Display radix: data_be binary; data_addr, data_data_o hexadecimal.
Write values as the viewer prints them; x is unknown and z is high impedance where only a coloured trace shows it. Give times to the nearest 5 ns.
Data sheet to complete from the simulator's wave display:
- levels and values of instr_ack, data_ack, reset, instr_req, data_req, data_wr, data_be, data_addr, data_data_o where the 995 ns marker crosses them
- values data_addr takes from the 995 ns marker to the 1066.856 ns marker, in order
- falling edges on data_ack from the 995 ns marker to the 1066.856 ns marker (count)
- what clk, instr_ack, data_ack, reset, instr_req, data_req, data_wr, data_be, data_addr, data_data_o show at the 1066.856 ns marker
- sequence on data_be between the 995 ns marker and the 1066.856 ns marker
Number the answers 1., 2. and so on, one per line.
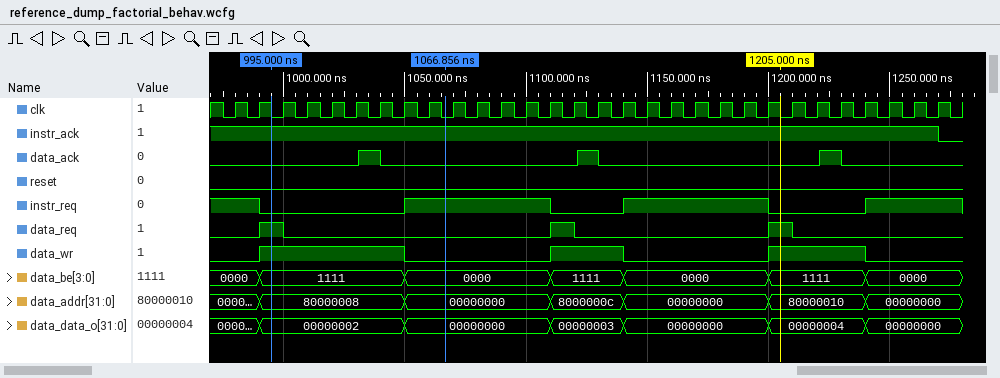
1. instr_ack=1, data_ack=0, reset=0, instr_req=0, data_req=1, data_wr=1, data_be=1111, data_addr=80000008, data_data_o=00000002
2. 80000008, 00000000
3. 1
4. clk=0, instr_ack=1, data_ack=0, reset=0, instr_req=1, data_req=0, data_wr=0, data_be=0000, data_addr=00000000, data_data_o=00000000
5. 1111, 0000
